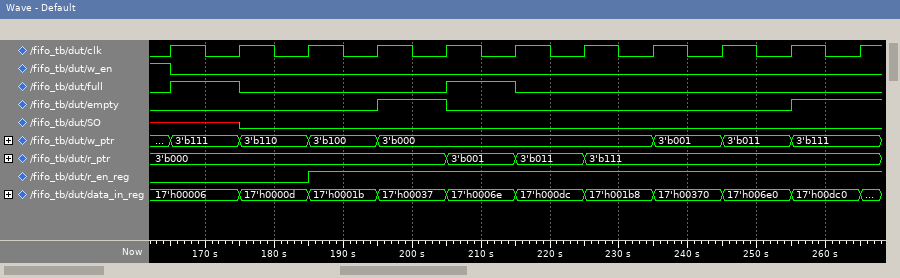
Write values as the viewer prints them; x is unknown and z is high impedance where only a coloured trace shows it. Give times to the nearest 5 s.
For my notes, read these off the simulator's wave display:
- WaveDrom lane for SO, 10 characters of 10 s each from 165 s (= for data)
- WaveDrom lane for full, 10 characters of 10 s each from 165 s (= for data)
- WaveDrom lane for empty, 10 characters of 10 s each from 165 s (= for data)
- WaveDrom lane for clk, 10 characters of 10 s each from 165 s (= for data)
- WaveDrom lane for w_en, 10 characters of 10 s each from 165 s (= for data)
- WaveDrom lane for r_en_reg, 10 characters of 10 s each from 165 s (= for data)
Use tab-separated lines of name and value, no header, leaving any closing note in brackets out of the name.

WaveDrom lane for SO, 10 characters of 10 s each from 165 s	{name: 'SO', wave: 'x0........'}
WaveDrom lane for full, 10 characters of 10 s each from 165 s	{name: 'full', wave: '10..10....'}
WaveDrom lane for empty, 10 characters of 10 s each from 165 s	{name: 'empty', wave: '0..10....1'}
WaveDrom lane for clk, 10 characters of 10 s each from 165 s	{name: 'clk', wave: 'p.........'}
WaveDrom lane for w_en, 10 characters of 10 s each from 165 s	{name: 'w_en', wave: '0.........'}
WaveDrom lane for r_en_reg, 10 characters of 10 s each from 165 s	{name: 'r_en_reg', wave: '0.1.......'}
